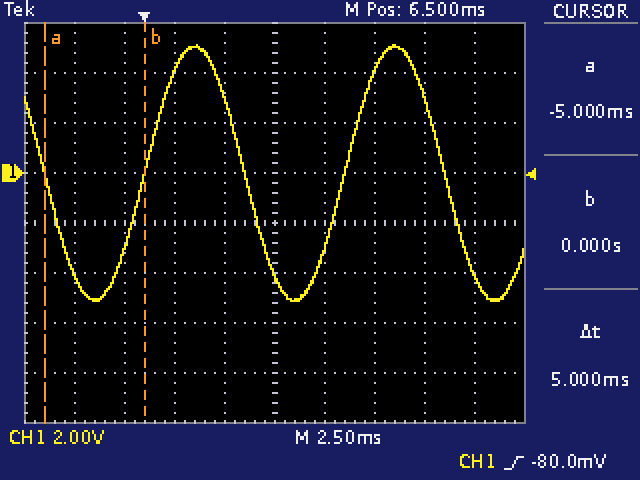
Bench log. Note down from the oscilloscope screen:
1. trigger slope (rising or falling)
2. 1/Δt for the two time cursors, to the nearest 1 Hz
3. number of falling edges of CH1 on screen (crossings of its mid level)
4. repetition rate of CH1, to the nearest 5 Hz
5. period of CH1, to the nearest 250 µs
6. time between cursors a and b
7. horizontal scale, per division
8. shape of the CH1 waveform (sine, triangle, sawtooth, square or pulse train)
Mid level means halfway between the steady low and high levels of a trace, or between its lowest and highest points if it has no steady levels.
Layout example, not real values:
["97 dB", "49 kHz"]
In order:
["rising", "200 Hz", "3", "100 Hz", "10.00 ms", "5 ms", "2.5 ms", "sine"]
